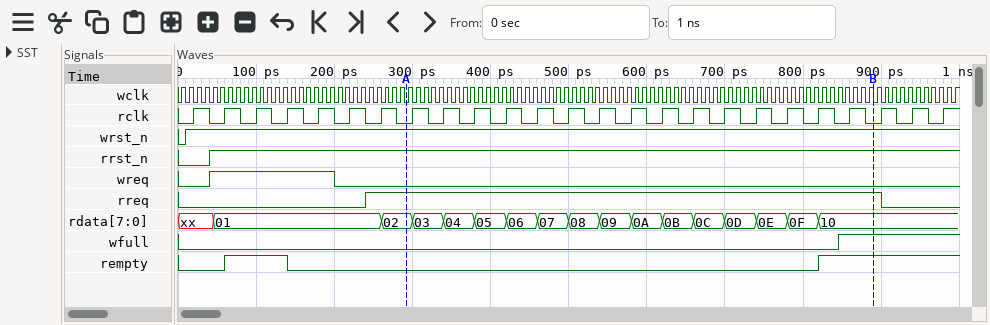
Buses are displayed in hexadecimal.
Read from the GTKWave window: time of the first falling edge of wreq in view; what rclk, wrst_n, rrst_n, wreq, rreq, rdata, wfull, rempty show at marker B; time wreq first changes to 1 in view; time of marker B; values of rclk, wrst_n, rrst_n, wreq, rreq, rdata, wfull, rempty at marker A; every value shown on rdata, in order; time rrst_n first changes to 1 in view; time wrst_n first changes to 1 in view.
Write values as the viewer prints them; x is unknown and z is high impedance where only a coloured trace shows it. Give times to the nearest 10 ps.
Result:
200 ps
rclk=0, wrst_n=1, rrst_n=1, wreq=0, rreq=1, rdata=10, wfull=1, rempty=1
40 ps
890 ps
rclk=0, wrst_n=1, rrst_n=1, wreq=0, rreq=1, rdata=02, wfull=0, rempty=0
xx, 01, 02, 03, 04, 05, 06, 07, 08, 09, 0A, 0B, 0C, 0D, 0E, 0F, 10
40 ps
10 ps
